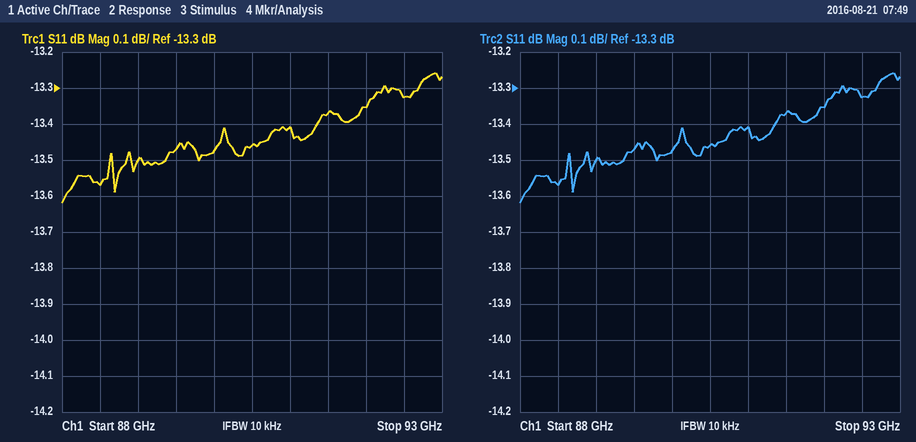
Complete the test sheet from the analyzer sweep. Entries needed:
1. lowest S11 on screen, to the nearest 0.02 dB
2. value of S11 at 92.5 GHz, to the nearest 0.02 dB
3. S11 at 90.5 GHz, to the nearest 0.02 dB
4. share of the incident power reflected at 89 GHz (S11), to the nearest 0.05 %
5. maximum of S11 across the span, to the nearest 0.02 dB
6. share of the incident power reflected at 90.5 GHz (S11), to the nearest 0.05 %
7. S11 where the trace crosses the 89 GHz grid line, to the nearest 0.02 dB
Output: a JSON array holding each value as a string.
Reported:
["-13.62 dB", "-13.32 dB", "-13.46 dB", "4.45 %", "-13.26 dB", "4.50 %", "-13.50 dB"]
